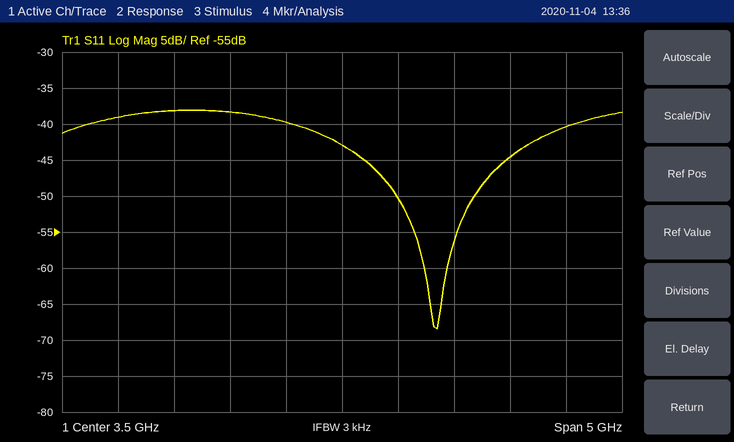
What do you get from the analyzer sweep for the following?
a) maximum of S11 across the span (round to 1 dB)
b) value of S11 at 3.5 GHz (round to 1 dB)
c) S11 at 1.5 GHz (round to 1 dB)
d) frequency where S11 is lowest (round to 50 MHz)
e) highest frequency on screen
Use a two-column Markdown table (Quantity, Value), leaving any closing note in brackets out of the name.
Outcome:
| Quantity | Value |
|---|---|
| maximum of S11 across the span | -38 dB |
| value of S11 at 3.5 GHz | -43 dB |
| S11 at 1.5 GHz | -39 dB |
| frequency where S11 is lowest | 4.35 GHz |
| highest frequency on screen | 6 GHz |
